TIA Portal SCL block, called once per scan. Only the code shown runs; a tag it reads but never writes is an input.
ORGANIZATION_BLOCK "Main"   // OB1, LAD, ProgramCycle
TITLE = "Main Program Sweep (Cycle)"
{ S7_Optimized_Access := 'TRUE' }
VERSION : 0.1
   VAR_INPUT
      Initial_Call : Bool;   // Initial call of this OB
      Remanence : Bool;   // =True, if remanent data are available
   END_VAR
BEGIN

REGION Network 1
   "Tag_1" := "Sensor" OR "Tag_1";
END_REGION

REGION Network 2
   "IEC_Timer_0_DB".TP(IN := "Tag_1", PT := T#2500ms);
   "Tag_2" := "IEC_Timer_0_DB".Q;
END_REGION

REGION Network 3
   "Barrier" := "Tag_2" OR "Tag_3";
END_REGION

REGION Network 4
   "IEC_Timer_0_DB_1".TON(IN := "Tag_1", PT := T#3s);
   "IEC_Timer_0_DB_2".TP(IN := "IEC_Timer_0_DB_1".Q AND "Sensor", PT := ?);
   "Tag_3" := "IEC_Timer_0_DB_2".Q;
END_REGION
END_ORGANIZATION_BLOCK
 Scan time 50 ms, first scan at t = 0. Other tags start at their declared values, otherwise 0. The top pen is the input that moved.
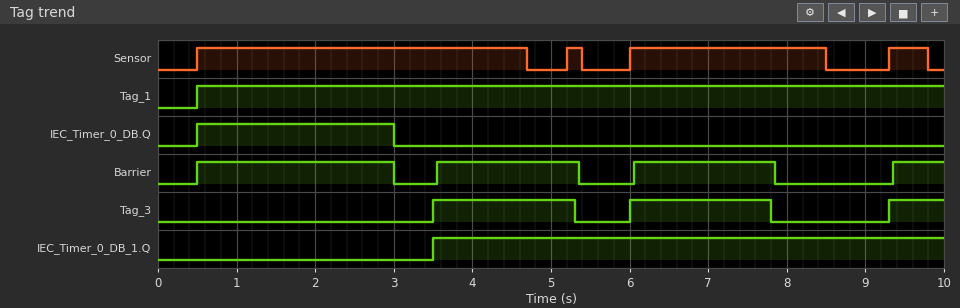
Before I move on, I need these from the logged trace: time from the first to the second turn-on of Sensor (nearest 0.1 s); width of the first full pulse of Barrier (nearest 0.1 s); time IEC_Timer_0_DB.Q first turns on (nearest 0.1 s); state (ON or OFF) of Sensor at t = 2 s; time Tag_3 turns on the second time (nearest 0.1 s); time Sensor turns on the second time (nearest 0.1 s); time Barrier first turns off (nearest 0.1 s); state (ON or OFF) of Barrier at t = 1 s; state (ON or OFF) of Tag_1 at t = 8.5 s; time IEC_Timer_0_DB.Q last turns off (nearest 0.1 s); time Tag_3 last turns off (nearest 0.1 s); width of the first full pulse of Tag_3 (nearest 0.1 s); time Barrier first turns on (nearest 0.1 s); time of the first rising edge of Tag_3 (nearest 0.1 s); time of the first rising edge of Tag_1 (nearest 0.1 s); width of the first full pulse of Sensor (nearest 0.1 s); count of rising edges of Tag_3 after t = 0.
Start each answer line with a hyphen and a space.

- 4.7 s
- 2.5 s
- 0.5 s
- ON
- 6.0 s
- 5.2 s
- 3.0 s
- ON
- ON
- 3.0 s
- 7.8 s
- 1.8 s
- 0.5 s
- 3.5 s
- 0.5 s
- 4.2 s
- 3
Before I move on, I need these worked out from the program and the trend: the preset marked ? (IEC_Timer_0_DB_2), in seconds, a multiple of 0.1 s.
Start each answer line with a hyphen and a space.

- 1.8 s
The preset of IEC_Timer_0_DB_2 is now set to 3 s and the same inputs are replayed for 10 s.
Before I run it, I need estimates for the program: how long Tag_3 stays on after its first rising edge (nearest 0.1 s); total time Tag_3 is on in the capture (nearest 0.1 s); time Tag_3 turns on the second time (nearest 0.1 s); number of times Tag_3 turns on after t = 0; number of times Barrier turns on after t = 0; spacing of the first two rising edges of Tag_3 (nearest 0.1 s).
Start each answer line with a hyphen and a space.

- 3.0 s
- 3.7 s
- 9.3 s
- 2
- 3
- 5.8 s
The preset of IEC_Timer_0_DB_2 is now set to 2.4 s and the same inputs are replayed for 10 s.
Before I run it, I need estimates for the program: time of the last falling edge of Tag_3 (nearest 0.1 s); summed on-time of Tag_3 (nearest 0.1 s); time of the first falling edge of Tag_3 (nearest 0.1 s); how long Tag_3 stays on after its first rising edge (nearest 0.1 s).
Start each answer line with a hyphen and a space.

- 8.4 s
- 5.5 s
- 5.9 s
- 2.4 s
